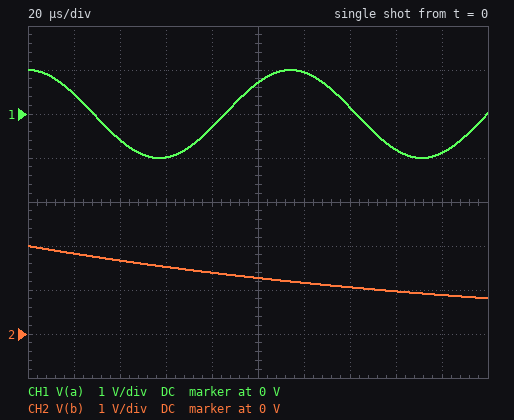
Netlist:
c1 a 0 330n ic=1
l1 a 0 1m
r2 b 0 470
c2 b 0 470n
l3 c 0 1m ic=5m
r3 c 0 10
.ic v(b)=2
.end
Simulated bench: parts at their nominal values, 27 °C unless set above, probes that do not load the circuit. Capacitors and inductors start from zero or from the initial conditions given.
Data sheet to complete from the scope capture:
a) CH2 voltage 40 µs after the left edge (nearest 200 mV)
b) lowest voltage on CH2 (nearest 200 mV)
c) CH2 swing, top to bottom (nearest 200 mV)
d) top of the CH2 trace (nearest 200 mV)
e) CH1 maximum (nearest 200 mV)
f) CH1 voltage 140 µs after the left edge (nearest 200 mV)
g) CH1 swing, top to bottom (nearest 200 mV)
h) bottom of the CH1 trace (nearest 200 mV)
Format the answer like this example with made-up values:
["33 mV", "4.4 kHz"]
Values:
["1.6 V", "800 mV", "1.2 V", "2.0 V", "1.0 V", "200 mV", "2.0 V", "-1.0 V"]
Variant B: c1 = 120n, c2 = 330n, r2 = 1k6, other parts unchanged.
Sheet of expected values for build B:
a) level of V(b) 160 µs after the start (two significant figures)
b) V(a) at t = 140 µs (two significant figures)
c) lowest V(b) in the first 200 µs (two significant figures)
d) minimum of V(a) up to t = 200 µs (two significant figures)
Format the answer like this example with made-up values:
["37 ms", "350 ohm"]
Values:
["1.5 V", "980 mV", "1.4 V", "-1.0 V"]
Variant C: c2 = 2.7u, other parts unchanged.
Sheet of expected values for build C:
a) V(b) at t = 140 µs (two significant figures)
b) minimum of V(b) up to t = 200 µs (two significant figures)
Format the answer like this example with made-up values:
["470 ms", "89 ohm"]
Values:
["1.8 V", "1.7 V"]
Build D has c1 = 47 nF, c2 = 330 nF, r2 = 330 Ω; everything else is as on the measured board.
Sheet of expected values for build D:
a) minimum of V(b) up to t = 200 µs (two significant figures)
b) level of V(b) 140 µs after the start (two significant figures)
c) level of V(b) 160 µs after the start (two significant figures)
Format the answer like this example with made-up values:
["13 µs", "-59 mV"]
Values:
["320 mV", "550 mV", "460 mV"]
